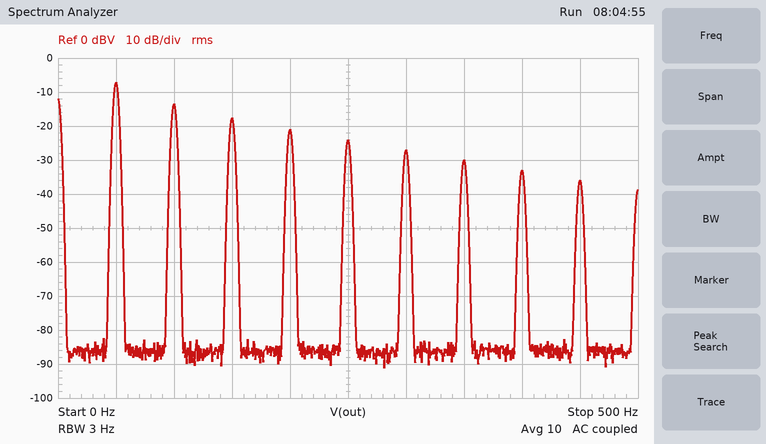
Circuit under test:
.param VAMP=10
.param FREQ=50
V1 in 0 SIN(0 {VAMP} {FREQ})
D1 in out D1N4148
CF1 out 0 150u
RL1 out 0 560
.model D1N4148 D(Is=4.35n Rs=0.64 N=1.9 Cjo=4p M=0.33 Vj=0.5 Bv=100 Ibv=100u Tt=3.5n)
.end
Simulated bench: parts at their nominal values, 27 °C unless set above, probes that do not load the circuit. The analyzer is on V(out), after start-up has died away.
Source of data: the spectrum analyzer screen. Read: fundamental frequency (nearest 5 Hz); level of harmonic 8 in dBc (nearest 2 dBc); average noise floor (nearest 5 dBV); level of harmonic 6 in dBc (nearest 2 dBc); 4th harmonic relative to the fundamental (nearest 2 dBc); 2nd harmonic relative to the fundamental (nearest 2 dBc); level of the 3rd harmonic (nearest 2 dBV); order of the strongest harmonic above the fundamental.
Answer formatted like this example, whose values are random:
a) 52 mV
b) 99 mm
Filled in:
a) 50 Hz
b) -26 dBc
c) -85 dBV
d) -20 dBc
e) -14 dBc
f) -6 dBc
g) -18 dBV
h) 2
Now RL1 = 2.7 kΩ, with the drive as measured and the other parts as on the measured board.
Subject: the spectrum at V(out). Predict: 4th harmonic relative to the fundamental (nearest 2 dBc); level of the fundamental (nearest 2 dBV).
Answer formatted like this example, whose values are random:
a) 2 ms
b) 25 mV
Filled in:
a) -12 dBc
b) -20 dBV
